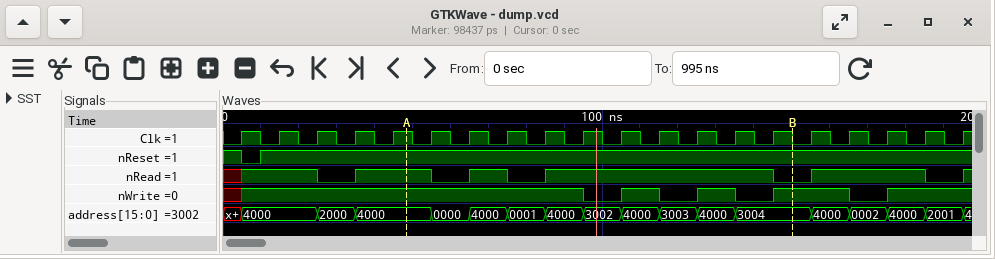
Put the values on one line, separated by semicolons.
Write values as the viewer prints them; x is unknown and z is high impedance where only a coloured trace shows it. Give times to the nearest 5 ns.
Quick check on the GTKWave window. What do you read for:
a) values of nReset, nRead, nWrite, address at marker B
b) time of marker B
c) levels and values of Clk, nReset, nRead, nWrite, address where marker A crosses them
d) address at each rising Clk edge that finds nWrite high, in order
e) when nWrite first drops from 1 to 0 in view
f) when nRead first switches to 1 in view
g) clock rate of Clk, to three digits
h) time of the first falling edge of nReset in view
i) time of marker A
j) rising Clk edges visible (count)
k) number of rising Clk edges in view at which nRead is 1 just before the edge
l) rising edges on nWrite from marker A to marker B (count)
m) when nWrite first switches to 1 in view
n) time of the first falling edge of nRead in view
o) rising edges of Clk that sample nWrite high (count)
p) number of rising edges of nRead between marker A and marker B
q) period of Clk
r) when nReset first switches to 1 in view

nReset=1, nRead=0, nWrite=1, address=3004; 150 ns; Clk=1, nReset=1, nRead=1, nWrite=1, address=4000; 4000, 4000, 2000, 4000, 4000, 0000, 4000, 0001, 4000, 4000, 4000, 3004, 4000, 4000, 2001; 95 ns; 5 ns; 100 MHz; 5 ns; 50 ns; 20; 14; 3; 5 ns; 25 ns; 15; 2; 10 ns; 10 ns
